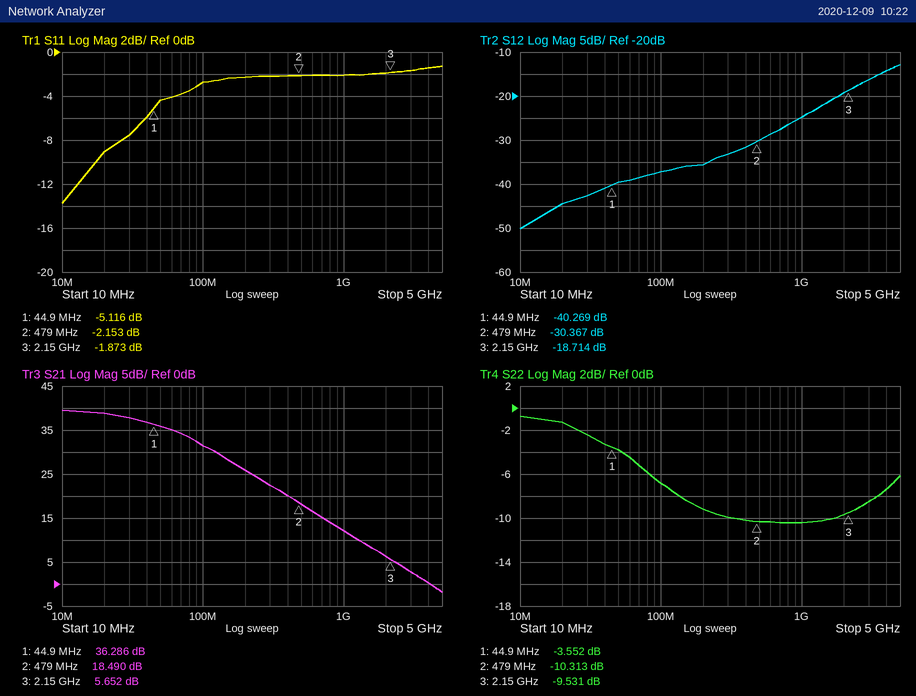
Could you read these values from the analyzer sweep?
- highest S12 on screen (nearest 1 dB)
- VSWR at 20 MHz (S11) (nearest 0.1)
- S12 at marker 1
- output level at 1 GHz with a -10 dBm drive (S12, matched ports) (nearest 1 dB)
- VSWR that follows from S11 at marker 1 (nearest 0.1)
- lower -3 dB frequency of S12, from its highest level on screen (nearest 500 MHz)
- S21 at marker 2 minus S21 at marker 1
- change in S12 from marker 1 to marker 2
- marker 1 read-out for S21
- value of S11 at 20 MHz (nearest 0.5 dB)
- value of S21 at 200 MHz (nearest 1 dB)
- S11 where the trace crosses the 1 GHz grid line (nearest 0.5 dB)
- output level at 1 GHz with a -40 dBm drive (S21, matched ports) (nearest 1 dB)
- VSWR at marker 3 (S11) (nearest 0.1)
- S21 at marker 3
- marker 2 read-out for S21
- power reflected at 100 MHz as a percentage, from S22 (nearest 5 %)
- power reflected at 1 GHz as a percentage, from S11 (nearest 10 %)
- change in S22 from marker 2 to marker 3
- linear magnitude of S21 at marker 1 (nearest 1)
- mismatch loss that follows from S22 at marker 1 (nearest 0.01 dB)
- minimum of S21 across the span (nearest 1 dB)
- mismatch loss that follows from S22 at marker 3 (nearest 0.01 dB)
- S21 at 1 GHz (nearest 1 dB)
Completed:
-13 dB
2.1
-40.269 dB
-35 dBm
3.5
3.0 GHz
-17.796 dB
9.902 dB
36.286 dB
-9.0 dB
26 dB
-2.0 dB
-28 dBm
9.3
5.652 dB
18.490 dB
20 %
60 %
0.782 dB
65
2.53 dB
-2 dB
0.51 dB
12 dB
